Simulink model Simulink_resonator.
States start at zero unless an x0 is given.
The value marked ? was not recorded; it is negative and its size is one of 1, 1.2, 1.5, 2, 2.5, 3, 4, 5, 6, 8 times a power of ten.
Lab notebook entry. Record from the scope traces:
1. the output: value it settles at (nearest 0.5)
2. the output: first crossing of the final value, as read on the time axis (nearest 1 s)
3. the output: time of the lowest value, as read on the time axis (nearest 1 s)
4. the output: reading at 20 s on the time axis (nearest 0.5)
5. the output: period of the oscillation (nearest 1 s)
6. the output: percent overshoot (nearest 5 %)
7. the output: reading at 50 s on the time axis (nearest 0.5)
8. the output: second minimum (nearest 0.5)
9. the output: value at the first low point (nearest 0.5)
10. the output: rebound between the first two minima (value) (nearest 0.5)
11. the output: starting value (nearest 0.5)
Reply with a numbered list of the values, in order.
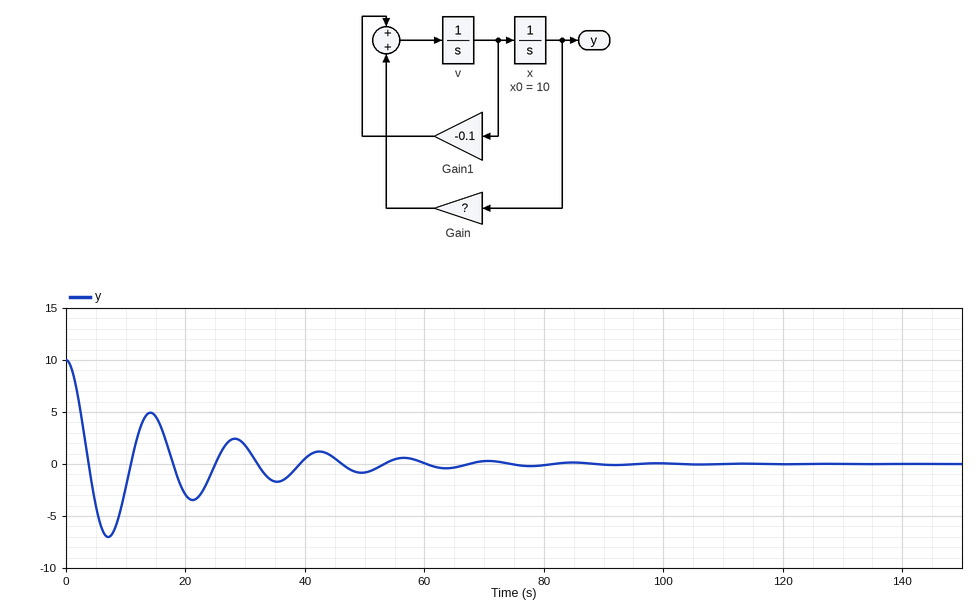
1. 0.0
2. 4 s
3. 7 s
4. -3.0
5. 14 s
6. 70 %
7. -1.0
8. -3.5
9. -7.0
10. 5.0
11. 10.0
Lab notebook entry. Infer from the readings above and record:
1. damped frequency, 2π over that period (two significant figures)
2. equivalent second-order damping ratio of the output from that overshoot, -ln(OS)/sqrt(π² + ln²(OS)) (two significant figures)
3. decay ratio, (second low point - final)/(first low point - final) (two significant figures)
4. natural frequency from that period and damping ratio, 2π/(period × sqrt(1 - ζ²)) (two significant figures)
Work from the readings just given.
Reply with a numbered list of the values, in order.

1. 0.45 rad/s
2. 0.11
3. 0.50
4. 0.45 rad/s
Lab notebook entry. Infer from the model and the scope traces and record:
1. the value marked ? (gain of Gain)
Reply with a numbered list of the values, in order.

1. -0.2
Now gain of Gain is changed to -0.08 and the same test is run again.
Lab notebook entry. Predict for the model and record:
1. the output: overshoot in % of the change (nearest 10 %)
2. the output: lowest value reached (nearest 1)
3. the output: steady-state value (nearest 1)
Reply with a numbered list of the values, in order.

1. 60 %
2. -6
3. 0
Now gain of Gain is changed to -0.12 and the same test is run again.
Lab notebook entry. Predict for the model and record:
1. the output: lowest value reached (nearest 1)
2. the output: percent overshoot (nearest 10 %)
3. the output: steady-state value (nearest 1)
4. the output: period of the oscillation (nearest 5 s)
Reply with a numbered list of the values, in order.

1. -6
2. 60 %
3. 0
4. 20 s
